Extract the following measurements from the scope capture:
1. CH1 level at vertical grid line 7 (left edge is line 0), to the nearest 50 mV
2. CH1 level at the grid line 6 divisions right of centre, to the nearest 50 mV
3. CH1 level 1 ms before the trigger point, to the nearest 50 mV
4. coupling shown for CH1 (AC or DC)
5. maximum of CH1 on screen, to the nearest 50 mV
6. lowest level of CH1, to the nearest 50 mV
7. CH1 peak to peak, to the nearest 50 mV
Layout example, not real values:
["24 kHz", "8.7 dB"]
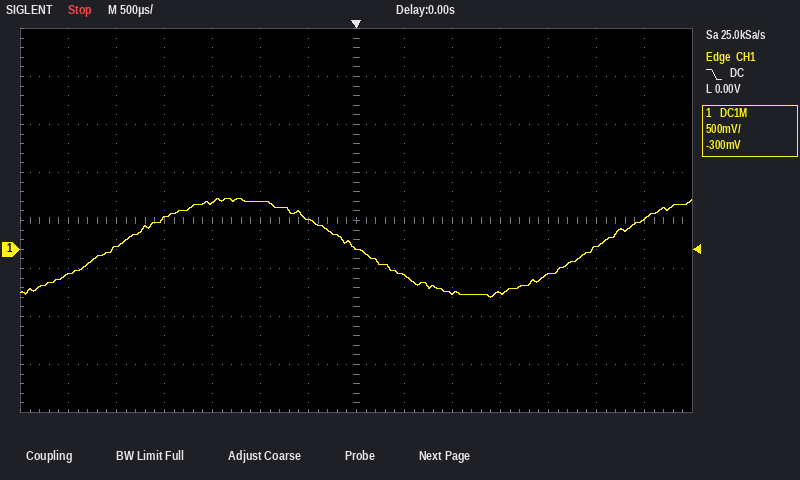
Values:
["0 mV", "300 mV", "500 mV", "DC", "550 mV", "-500 mV", "1.05 V"]
